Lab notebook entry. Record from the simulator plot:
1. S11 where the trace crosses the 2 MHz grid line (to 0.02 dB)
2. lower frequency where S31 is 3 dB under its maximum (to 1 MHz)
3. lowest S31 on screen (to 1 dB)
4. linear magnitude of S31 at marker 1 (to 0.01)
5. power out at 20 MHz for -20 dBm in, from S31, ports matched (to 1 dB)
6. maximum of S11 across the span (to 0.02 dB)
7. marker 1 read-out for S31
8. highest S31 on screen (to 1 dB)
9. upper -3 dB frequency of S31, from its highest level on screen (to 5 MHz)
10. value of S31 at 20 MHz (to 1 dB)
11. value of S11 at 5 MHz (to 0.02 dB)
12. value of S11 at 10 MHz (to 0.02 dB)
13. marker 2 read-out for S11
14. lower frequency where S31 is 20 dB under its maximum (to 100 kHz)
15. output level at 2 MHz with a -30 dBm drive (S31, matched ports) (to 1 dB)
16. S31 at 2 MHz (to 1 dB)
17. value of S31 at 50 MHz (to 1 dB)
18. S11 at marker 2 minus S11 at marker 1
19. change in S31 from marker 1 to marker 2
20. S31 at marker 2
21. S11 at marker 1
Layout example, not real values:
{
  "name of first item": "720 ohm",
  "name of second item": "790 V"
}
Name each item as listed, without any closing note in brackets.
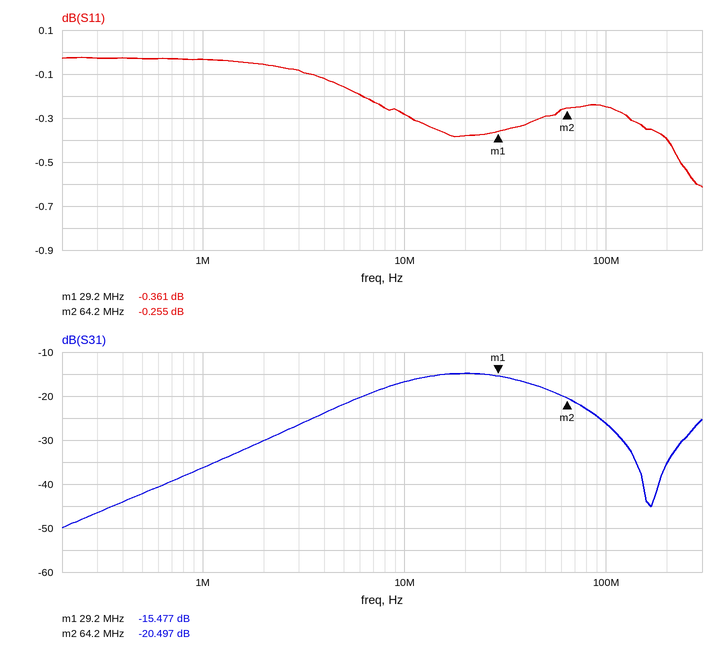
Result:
{
  "S11 where the trace crosses the 2 MHz grid line": "-0.06 dB",
  "lower frequency where S31 is 3 dB under its maximum": "8 MHz",
  "lowest S31 on screen": "-50 dB",
  "linear magnitude of S31 at marker 1": "0.17",
  "power out at 20 MHz for -20 dBm in, from S31, ports matched": "-35 dBm",
  "maximum of S11 across the span": "-0.02 dB",
  "marker 1 read-out for S31": "-15.477 dB",
  "highest S31 on screen": "-15 dB",
  "upper -3 dB frequency of S31, from its highest level on screen": "45 MHz",
  "value of S31 at 20 MHz": "-15 dB",
  "value of S11 at 5 MHz": "-0.16 dB",
  "value of S11 at 10 MHz": "-0.28 dB",
  "marker 2 read-out for S11": "-0.255 dB",
  "lower frequency where S31 is 20 dB under its maximum": "1.2 MHz",
  "output level at 2 MHz with a -30 dBm drive (S31, matched ports)": "-60 dBm",
  "S31 at 2 MHz": "-30 dB",
  "value of S31 at 50 MHz": "-18 dB",
  "S11 at marker 2 minus S11 at marker 1": "0.106 dB",
  "change in S31 from marker 1 to marker 2": "-5.020 dB",
  "S31 at marker 2": "-20.497 dB",
  "S11 at marker 1": "-0.361 dB"
}
